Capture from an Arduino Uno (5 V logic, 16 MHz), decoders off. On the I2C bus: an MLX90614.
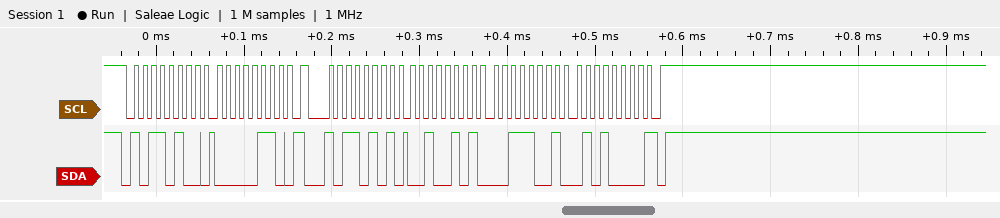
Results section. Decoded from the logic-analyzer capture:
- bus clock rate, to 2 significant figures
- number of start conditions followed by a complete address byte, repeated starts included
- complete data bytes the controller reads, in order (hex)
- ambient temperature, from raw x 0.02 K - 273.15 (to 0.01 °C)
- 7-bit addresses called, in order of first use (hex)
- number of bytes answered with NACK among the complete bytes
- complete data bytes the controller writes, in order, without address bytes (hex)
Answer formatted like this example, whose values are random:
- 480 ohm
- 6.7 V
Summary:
- 100 kHz
- 2
- 25 39 50
- 19.43 °C
- 0x5A
- 1
- 06
